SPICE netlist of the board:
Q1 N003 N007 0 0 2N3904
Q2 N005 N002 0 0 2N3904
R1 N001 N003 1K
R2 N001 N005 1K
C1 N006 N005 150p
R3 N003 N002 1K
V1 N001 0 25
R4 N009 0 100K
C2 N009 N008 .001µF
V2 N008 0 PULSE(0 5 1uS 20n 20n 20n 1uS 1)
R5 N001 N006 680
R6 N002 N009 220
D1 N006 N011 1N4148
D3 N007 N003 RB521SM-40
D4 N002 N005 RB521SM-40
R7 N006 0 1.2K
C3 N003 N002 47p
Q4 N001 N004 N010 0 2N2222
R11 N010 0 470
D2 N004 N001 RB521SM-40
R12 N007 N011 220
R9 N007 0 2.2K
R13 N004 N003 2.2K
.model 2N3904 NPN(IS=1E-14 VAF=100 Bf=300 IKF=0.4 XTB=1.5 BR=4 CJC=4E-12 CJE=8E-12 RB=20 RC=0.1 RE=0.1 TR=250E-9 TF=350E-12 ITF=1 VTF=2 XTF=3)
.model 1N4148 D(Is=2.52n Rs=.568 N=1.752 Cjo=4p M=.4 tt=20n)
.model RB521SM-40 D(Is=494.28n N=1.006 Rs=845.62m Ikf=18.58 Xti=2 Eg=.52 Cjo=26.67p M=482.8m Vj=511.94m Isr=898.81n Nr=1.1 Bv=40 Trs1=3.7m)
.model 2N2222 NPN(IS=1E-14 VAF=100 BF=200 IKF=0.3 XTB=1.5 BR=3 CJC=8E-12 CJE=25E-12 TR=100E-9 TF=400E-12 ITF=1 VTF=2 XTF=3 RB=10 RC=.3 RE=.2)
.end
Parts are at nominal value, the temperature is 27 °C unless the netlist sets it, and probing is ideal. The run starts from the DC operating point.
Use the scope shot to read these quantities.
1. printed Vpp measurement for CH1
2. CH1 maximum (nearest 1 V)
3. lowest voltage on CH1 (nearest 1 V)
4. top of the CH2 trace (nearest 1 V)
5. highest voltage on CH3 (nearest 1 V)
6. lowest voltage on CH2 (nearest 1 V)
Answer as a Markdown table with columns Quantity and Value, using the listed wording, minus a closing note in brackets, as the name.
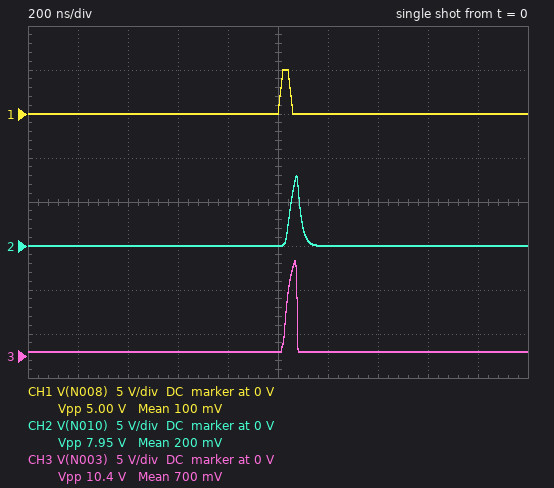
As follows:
| Quantity | Value |
|---|---|
| printed Vpp measurement for CH1 | 5.00 V |
| CH1 maximum | 5 V |
| lowest voltage on CH1 | 0 V |
| top of the CH2 trace | 8 V |
| highest voltage on CH3 | 11 V |
| lowest voltage on CH2 | 0 V |
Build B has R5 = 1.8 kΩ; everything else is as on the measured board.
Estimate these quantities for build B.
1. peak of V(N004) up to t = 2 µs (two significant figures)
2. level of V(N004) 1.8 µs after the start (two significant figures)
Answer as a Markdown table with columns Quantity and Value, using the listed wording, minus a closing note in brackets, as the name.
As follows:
| Quantity | Value |
|---|---|
| peak of V(N004) up to t = 2 µs | 10 V |
| level of V(N004) 1.8 µs after the start | 500 mV |
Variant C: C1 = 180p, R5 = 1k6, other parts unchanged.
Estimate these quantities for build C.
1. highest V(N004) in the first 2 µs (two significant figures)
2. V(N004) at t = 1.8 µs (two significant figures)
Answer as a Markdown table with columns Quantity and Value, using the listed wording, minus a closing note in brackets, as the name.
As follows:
| Quantity | Value |
|---|---|
| highest V(N004) in the first 2 µs | 11 V |
| V(N004) at t = 1.8 µs | 500 mV |
